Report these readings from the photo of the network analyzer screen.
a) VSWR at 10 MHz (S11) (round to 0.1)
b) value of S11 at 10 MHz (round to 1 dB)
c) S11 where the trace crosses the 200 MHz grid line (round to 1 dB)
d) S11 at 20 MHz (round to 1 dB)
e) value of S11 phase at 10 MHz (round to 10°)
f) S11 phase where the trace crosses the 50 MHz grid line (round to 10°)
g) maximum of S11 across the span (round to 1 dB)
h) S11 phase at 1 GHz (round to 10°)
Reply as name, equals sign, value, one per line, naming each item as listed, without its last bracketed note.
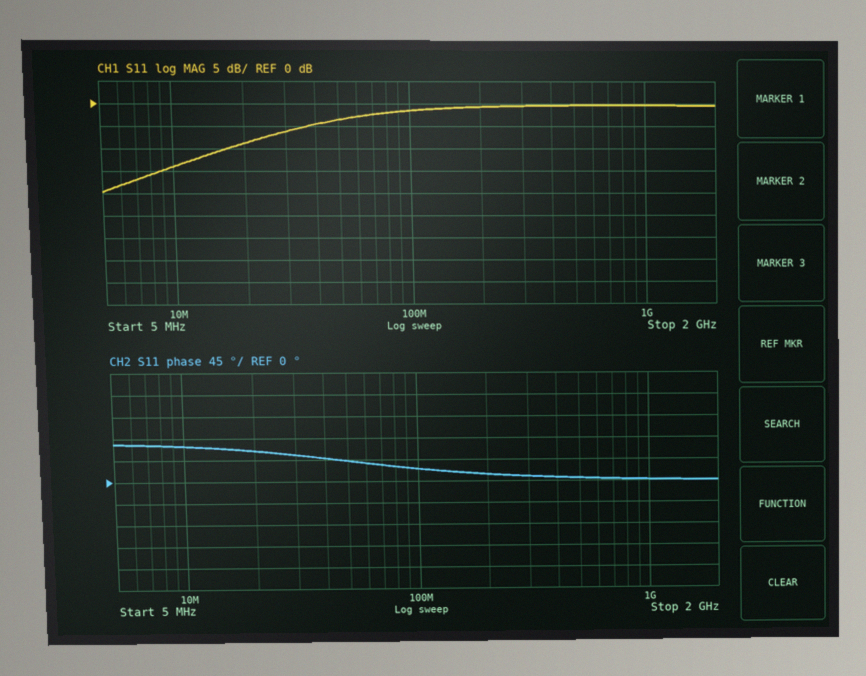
VSWR at 10 MHz (S11) = 1.5
value of S11 at 10 MHz = -14 dB
S11 where the trace crosses the 200 MHz grid line = -1 dB
S11 at 20 MHz = -9 dB
value of S11 phase at 10 MHz = 70°
S11 phase where the trace crosses the 50 MHz grid line = 40°
maximum of S11 across the span = 0 dB
S11 phase at 1 GHz = 0°
